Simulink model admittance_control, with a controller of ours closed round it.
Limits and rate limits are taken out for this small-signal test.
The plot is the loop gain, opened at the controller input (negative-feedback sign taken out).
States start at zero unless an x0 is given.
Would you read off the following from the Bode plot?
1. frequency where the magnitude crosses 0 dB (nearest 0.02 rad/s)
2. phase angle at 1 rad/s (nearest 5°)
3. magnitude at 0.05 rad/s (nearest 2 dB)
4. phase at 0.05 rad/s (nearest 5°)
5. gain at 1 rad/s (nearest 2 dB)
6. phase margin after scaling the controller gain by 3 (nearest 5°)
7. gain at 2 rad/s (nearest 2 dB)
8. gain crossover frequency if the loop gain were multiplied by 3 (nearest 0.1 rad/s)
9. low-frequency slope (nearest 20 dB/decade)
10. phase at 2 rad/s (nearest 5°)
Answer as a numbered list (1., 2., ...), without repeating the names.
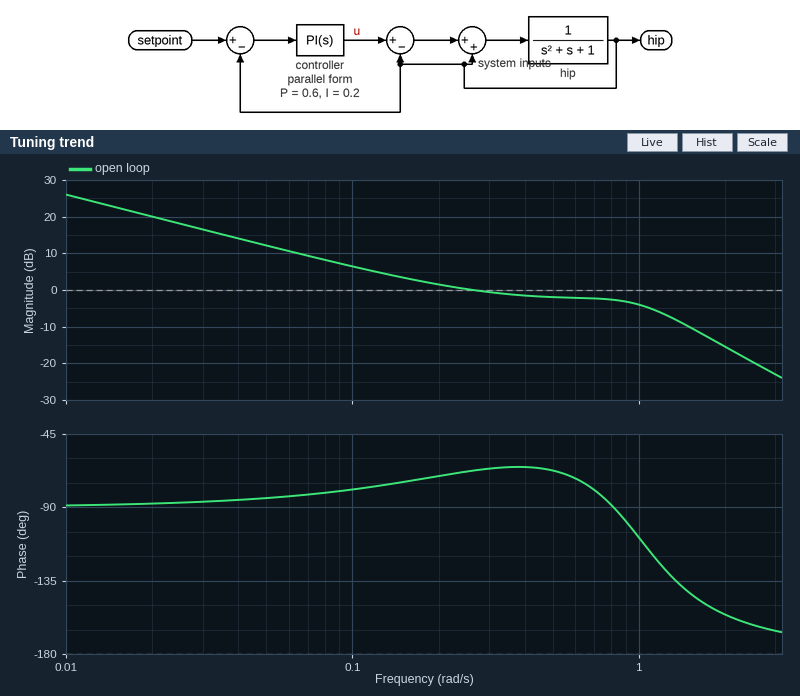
1. 0.26 rad/s
2. -110°
3. 12 dB
4. -85°
5. -4 dB
6. 40°
7. -16 dB
8. 1.5 rad/s
9. -20 dB/decade
10. -155°
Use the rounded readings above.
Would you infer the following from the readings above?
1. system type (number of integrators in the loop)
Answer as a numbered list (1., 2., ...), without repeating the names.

1. 1
